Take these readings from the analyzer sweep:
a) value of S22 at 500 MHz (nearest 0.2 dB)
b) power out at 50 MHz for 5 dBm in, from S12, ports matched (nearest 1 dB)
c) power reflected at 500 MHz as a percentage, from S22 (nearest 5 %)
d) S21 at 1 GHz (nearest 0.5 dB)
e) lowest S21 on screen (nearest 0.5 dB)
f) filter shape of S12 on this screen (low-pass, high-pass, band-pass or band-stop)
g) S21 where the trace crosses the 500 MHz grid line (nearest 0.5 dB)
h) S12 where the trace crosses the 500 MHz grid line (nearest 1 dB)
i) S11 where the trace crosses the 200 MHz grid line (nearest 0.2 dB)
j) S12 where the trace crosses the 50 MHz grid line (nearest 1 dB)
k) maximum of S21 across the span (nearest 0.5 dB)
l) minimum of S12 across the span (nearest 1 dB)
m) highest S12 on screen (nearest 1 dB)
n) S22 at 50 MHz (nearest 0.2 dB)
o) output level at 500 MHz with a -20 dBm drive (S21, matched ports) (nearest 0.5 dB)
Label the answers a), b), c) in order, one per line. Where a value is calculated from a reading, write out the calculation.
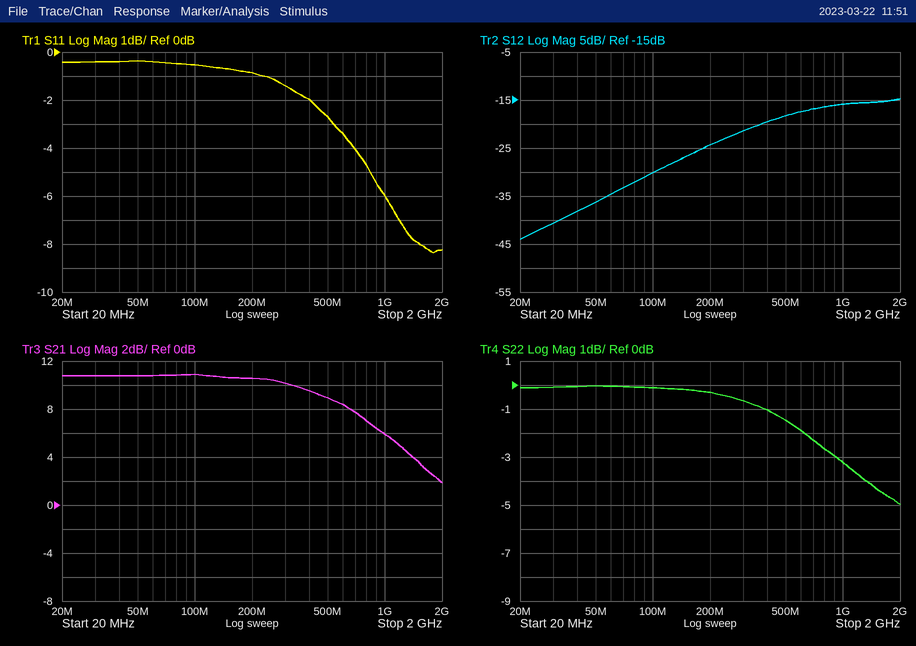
a) -1.4 dB
b) 5 dBm + (-36 dB) = -31 dBm
c) 10^(-1.4/10) ≈ 72.4 %, so 70 % to the nearest 5 %
d) 6.0 dB
e) 2.0 dB
f) high-pass
g) 9.0 dB
h) -18 dB
i) -0.8 dB
j) -36 dB
k) 11.0 dB
l) -44 dB
m) -15 dB
n) 0.0 dB
o) -20 dBm + (9.0 dB) = -11.0 dBm
